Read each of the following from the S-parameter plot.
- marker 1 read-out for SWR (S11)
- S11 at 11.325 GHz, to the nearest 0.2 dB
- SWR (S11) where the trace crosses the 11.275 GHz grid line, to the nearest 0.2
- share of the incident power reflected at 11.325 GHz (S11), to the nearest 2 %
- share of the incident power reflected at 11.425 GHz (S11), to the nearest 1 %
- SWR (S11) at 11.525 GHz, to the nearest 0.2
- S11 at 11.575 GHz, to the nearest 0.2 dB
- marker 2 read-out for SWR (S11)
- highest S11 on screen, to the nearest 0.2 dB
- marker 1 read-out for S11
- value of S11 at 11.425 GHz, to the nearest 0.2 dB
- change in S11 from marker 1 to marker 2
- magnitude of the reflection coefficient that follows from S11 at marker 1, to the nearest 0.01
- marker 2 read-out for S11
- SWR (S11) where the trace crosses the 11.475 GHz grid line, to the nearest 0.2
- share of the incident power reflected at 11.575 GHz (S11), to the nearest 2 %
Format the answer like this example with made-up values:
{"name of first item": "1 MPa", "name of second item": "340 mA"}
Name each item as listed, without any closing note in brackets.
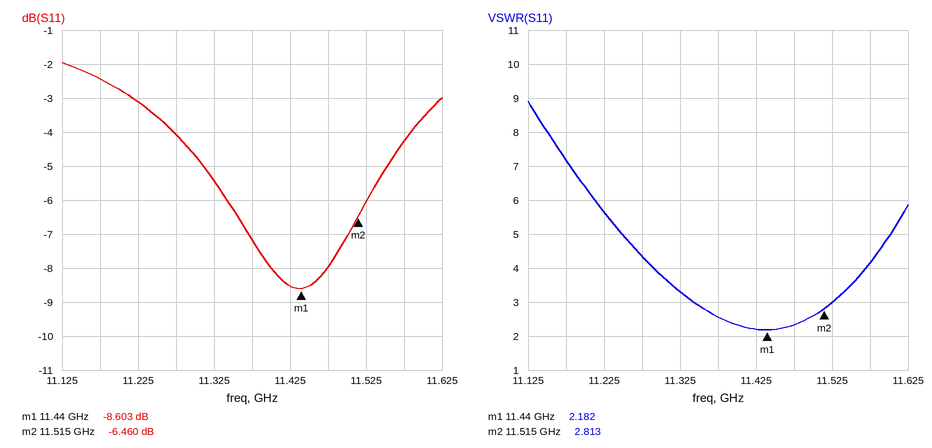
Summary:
{"marker 1 read-out for SWR": "2.182", "S11 at 11.325 GHz, to the nearest 0.2 dB": "-5.4 dB", "SWR (S11) where the trace crosses the 11.275 GHz grid line, to the nearest 0.2": "4.4", "share of the incident power reflected at 11.325 GHz (S11), to the nearest 2 %": "28 %", "share of the incident power reflected at 11.425 GHz (S11), to the nearest 1 %": "14 %", "SWR (S11) at 11.525 GHz, to the nearest 0.2": "3.0", "S11 at 11.575 GHz, to the nearest 0.2 dB": "-4.2 dB", "marker 2 read-out for SWR": "2.813", "highest S11 on screen, to the nearest 0.2 dB": "-2.0 dB", "marker 1 read-out for S11": "-8.603 dB", "value of S11 at 11.425 GHz, to the nearest 0.2 dB": "-8.6 dB", "change in S11 from marker 1 to marker 2": "2.143 dB", "magnitude of the reflection coefficient that follows from S11 at marker 1, to the nearest 0.01": "0.37", "marker 2 read-out for S11": "-6.460 dB", "SWR (S11) where the trace crosses the 11.475 GHz grid line, to the nearest 0.2": "2.4", "share of the incident power reflected at 11.575 GHz (S11), to the nearest 2 %": "38 %"}
